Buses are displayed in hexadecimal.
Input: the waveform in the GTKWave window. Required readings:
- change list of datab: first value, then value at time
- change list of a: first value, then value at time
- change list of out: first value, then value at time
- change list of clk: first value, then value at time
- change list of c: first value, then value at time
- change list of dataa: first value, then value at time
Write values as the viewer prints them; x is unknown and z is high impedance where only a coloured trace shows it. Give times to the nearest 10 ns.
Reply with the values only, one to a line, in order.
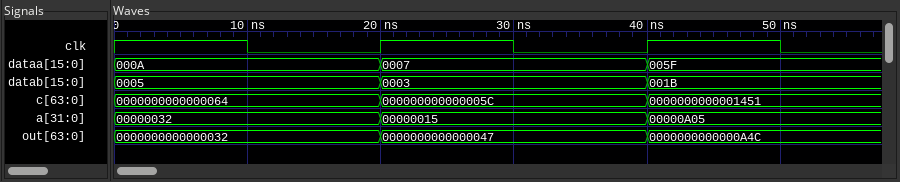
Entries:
0005, 0003 at 20 ns, 001B at 40 ns
00000032, 00000015 at 20 ns, 00000A05 at 40 ns
0000000000000032, 0000000000000047 at 20 ns, 0000000000000A4C at 40 ns
1, 0 at 10 ns, 1 at 20 ns, 0 at 30 ns, 1 at 40 ns, 0 at 50 ns
0000000000000064, 000000000000005C at 20 ns, 0000000000001451 at 40 ns
000A, 0007 at 20 ns, 005F at 40 ns
